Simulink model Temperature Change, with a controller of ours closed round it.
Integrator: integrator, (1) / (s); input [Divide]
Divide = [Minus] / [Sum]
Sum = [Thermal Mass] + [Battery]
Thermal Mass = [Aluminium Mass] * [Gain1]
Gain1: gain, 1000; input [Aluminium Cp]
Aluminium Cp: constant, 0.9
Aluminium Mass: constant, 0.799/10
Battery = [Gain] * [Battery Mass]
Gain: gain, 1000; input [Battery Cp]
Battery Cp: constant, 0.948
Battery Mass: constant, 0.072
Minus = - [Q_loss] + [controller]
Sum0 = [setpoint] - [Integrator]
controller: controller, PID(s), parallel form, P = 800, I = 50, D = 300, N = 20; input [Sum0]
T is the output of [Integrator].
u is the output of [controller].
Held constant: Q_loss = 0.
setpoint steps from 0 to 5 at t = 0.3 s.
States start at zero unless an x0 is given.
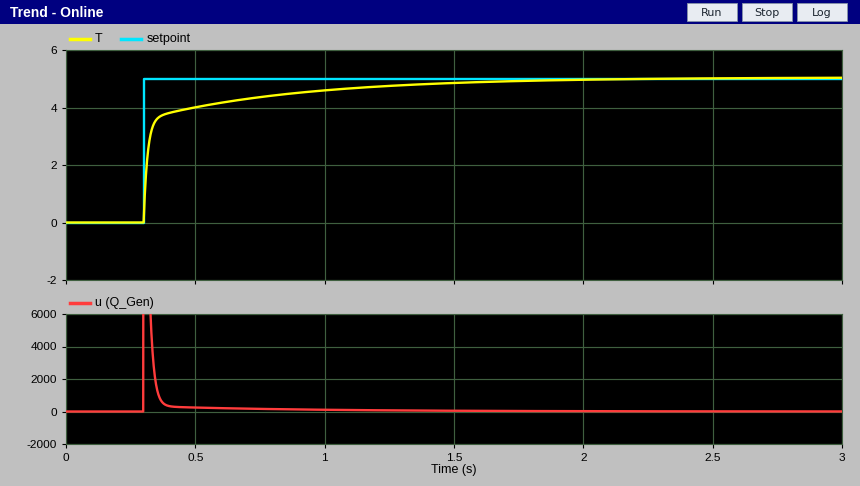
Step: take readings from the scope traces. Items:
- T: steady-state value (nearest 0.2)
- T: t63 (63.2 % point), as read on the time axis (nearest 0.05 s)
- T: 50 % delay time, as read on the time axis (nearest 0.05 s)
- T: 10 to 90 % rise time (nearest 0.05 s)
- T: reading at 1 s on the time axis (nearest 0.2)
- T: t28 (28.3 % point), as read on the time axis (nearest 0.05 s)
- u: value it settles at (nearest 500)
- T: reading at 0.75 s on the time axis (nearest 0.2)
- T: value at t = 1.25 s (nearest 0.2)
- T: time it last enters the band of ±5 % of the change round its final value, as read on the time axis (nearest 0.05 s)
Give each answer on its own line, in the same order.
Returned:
5.0
0.35 s
0.30 s
0.60 s
4.6
0.30 s
0
4.4
4.8
1.30 s
